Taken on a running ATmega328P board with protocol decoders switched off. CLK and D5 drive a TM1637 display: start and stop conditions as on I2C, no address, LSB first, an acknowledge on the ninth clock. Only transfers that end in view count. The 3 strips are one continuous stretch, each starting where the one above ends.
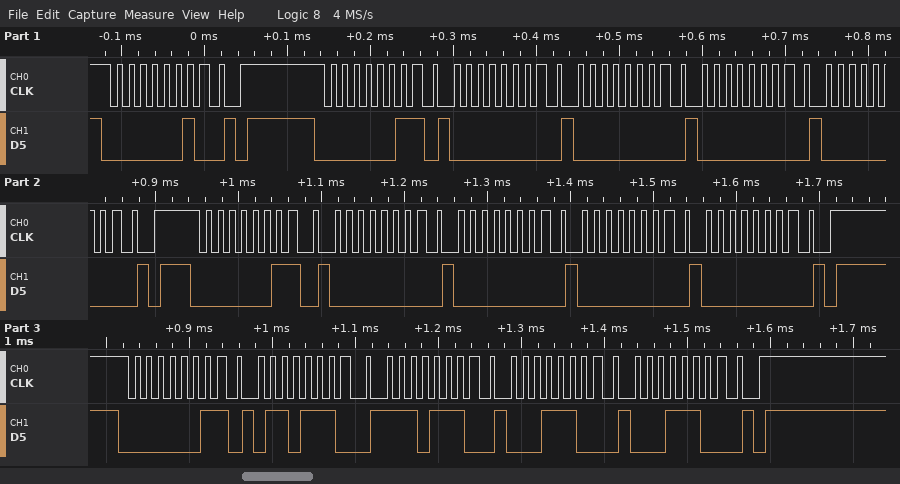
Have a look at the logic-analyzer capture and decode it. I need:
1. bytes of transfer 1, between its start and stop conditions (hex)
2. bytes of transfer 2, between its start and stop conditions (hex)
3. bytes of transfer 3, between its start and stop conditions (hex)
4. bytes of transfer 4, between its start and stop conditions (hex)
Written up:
40
C0 00 00 00 00
C0 00 00 00 00
C0 76 77 38 38
